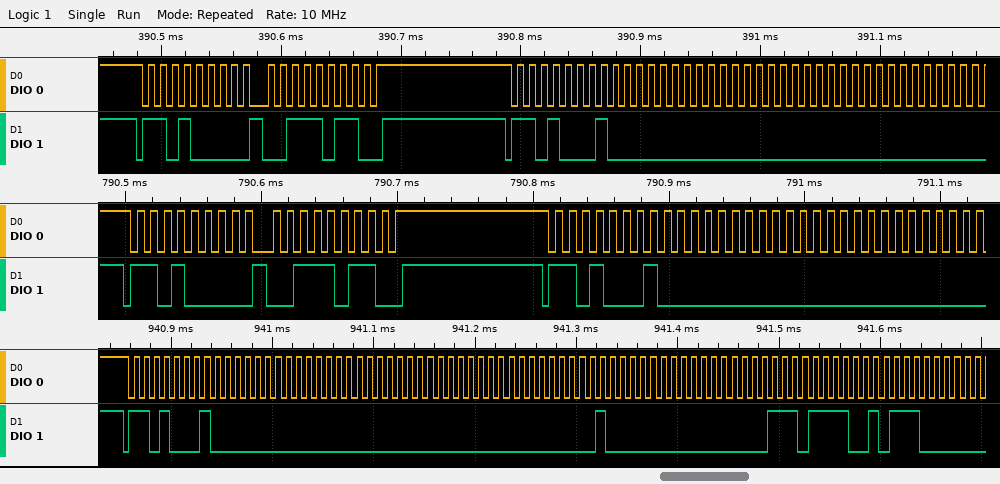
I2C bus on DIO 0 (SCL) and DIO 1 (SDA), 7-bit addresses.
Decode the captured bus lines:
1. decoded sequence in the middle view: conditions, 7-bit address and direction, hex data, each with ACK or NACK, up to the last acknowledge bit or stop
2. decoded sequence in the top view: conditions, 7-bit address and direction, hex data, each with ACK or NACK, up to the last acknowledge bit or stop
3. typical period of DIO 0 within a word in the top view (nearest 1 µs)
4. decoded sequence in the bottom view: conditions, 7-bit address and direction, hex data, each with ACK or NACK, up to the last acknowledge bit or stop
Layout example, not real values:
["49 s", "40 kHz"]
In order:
["start, address 68 write ACK, 3B ACK, stop, start, address 68 read ACK, 00 ACK, 00 ACK", "start, address 68 write ACK, 3B ACK, stop, start, address 68 read ACK, 00 ACK, 00 ACK, 00 ACK", "10 µs", "start, address 68 read ACK, 00 ACK, 00 ACK, 00 ACK, 00 ACK, 40 ACK, 00 ACK, EF ACK, 5C ACK"]
